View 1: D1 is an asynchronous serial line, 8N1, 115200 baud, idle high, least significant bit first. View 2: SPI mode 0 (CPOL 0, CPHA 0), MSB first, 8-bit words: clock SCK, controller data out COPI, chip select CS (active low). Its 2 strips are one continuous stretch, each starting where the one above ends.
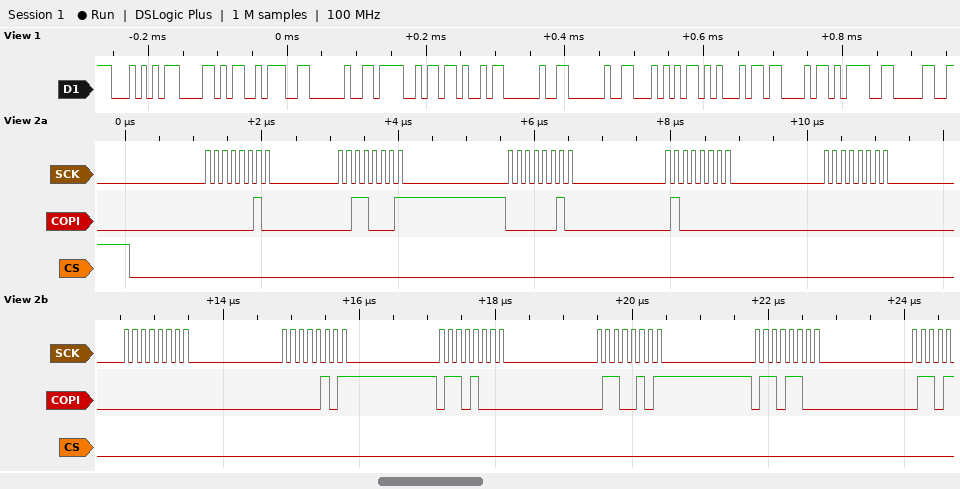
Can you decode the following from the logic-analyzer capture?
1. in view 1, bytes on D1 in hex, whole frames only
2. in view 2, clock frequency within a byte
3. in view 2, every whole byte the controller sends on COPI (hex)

54 58 3A 20 4F 4B 20 20 54 45 43 3D 30
8 MHz
02 31 02 40 00 00 05 68 65 6C
